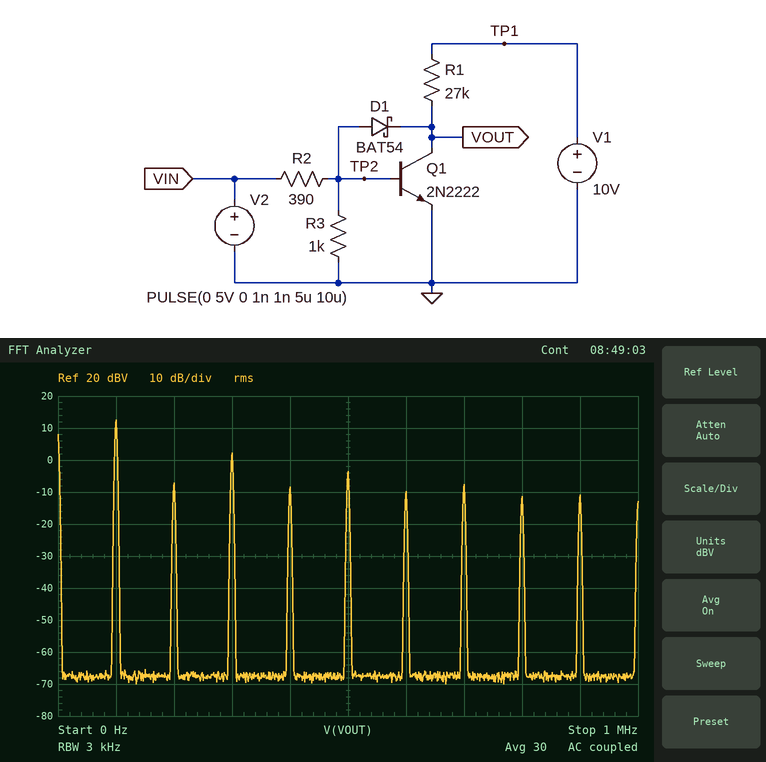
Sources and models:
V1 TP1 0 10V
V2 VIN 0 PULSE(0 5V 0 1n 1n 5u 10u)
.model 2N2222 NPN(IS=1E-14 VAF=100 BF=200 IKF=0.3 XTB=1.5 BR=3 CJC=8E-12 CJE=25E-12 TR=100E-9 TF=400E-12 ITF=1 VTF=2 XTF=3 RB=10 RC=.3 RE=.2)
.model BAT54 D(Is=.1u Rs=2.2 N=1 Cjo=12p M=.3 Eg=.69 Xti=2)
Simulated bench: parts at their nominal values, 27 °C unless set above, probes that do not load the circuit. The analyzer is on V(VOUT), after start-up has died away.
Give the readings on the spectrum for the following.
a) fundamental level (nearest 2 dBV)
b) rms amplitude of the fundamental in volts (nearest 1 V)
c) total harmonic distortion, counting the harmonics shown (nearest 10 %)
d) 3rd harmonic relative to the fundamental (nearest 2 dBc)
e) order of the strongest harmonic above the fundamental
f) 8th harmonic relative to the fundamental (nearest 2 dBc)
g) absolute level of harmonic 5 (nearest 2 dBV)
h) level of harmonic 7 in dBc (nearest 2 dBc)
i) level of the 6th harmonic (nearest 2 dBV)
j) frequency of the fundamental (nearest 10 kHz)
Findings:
12 dBV
4 V
40 %
-10 dBc
3
-24 dBc
-4 dBV
-20 dBc
-10 dBV
100 kHz
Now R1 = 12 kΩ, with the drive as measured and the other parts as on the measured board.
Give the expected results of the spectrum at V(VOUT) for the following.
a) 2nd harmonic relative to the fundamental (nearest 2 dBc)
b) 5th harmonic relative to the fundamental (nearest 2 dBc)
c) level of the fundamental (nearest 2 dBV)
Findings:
-26 dBc
-14 dBc
12 dBV
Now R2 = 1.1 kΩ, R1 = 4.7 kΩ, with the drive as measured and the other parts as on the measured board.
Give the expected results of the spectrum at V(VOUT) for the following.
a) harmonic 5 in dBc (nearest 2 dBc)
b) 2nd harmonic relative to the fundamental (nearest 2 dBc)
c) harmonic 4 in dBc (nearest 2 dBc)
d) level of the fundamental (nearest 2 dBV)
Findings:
-14 dBc
-36 dBc
-36 dBc
12 dBV
